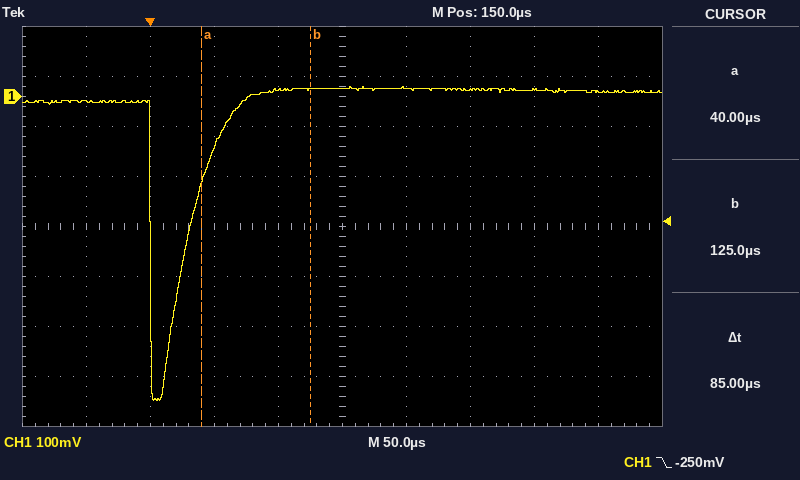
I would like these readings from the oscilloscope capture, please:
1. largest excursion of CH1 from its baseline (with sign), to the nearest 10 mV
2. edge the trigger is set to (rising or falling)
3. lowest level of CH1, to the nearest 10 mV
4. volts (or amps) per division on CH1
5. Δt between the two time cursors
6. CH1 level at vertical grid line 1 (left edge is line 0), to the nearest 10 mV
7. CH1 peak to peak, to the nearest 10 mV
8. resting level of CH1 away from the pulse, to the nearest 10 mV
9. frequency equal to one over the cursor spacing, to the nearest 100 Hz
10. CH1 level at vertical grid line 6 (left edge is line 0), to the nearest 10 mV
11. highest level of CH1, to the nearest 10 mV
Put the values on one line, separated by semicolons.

-620 mV; falling; -610 mV; 100 mV; 85 µs; -10 mV; 630 mV; 10 mV; 11.8 kHz; 20 mV; 20 mV
